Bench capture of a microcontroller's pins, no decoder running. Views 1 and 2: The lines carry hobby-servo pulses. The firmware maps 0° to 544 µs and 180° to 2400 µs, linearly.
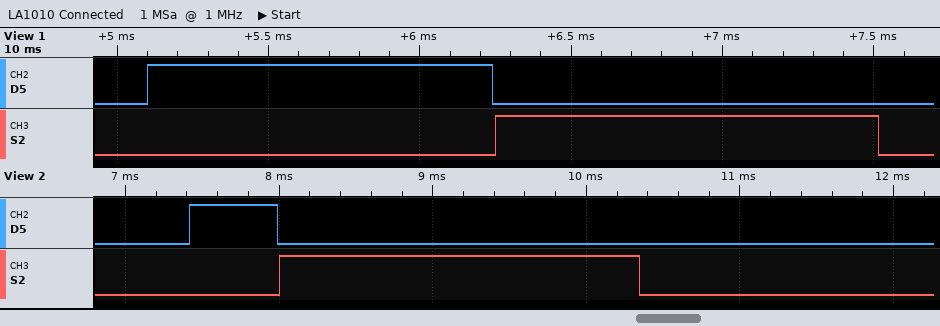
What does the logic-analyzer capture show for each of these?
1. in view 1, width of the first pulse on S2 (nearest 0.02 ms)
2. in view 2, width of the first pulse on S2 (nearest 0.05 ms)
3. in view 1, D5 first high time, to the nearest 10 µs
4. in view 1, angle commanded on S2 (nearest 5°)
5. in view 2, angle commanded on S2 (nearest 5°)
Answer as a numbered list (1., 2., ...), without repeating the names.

1. 1.26 ms
2. 2.35 ms
3. 1140 µs
4. 70°
5. 175°
